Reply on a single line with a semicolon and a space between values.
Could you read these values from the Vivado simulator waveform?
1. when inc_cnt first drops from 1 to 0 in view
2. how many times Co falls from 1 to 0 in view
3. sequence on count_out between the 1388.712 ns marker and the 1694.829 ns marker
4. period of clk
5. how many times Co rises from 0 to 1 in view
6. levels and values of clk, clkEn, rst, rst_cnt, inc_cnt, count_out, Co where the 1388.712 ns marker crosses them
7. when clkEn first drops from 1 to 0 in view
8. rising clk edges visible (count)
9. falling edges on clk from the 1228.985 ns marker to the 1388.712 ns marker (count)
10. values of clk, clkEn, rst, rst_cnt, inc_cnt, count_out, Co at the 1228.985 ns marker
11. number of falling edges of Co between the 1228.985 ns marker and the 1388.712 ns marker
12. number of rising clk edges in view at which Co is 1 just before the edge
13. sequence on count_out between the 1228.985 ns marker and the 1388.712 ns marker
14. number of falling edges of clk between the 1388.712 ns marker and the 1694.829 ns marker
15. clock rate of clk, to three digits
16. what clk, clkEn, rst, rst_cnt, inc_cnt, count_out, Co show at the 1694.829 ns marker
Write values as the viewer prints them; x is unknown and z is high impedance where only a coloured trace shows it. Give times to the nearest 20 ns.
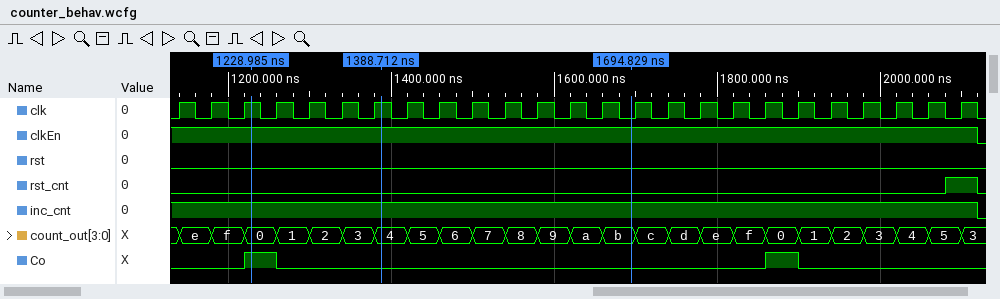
2120 ns; 2; 4, 5, 6, 7, 8, 9, a, b; 40 ns; 2; clk=1, clkEn=1, rst=0, rst_cnt=0, inc_cnt=1, count_out=4, Co=0; 2120 ns; 25; 4; clk=1, clkEn=1, rst=0, rst_cnt=0, inc_cnt=1, count_out=0, Co=1; 1; 2; 0, 1, 2, 3, 4; 8; 25.0 MHz; clk=0, clkEn=1, rst=0, rst_cnt=0, inc_cnt=1, count_out=b, Co=0
